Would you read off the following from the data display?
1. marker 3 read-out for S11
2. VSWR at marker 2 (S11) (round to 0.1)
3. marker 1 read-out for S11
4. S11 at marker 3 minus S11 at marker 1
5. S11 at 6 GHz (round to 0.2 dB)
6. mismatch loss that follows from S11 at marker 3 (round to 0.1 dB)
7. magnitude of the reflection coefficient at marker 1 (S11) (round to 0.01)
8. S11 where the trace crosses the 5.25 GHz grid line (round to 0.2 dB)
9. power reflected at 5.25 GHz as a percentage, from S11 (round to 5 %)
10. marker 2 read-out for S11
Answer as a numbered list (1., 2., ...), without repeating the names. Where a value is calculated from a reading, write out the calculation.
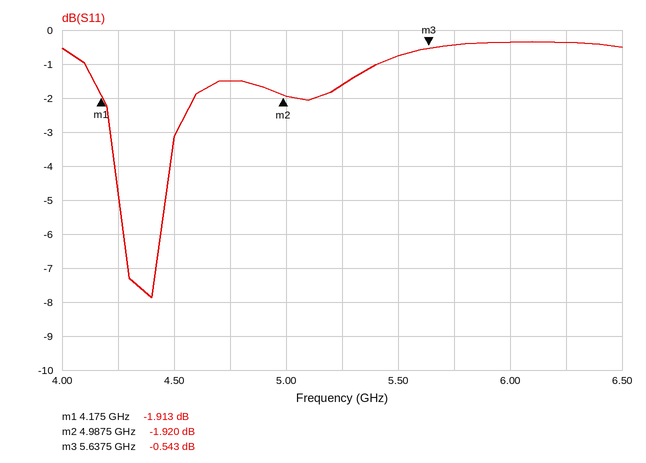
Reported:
1. -0.543 dB
2. (1 + 0.8017)/(1 − 0.8017) ≈ 9.1
3. -1.913 dB
4. -0.543 − (-1.913) = 1.370 dB
5. -0.4 dB
6. −10 log10(1 − 10^(-0.543/10)) ≈ 9.3 dB
7. 10^(-1.913/20) ≈ 0.80
8. -1.6 dB
9. 10^(-1.6/10) ≈ 69.2 %, so 70 % to the nearest 5 %
10. -1.920 dB
